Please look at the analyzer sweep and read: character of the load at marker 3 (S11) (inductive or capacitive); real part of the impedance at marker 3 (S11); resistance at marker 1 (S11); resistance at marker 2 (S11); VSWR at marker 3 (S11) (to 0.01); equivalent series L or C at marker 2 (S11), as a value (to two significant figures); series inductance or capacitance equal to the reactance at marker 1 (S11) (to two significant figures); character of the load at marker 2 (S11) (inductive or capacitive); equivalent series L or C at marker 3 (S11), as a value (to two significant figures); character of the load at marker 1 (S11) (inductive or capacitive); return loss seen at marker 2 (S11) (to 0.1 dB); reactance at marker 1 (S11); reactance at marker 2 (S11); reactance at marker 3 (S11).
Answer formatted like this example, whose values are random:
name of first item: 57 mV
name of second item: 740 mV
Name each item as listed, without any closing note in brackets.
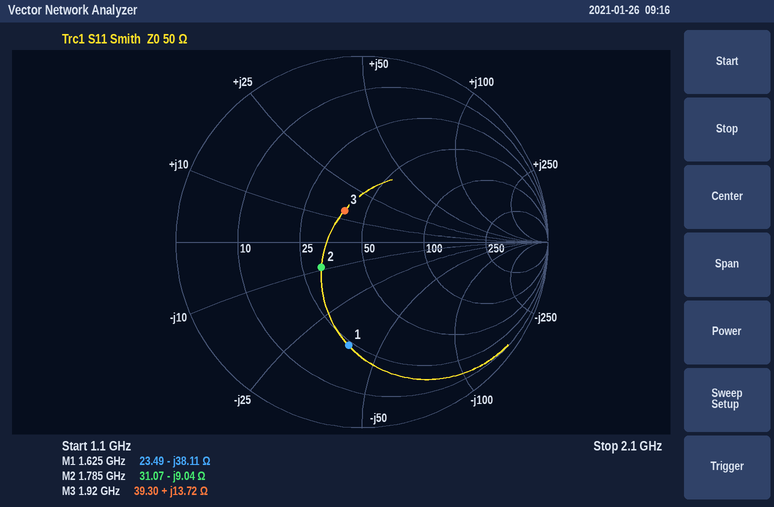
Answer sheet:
character of the load at marker 3 (S11): inductive
real part of the impedance at marker 3: 39.30 Ω
resistance at marker 1: 23.49 Ω
resistance at marker 2: 31.07 Ω
VSWR at marker 3 (S11): 1.48
equivalent series L or C at marker 2 (S11), as a value: 9.9 pF
series inductance or capacitance equal to the reactance at marker 1 (S11): 2.6 pF
character of the load at marker 2 (S11): capacitive
equivalent series L or C at marker 3 (S11), as a value: 1.1 nH
character of the load at marker 1 (S11): capacitive
return loss seen at marker 2 (S11): 11.8 dB
reactance at marker 1: -38.11 Ω
reactance at marker 2: -9.04 Ω
reactance at marker 3: +13.72 Ω
